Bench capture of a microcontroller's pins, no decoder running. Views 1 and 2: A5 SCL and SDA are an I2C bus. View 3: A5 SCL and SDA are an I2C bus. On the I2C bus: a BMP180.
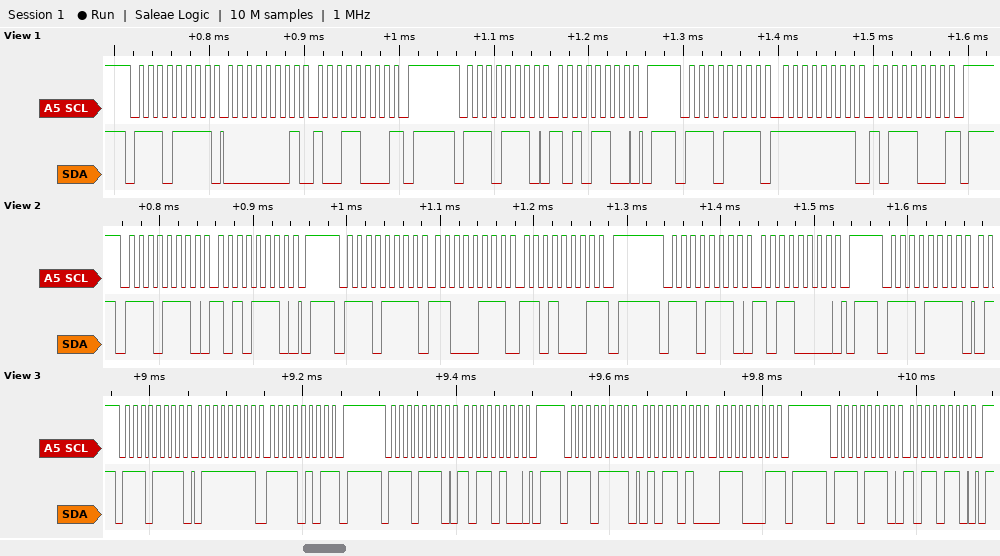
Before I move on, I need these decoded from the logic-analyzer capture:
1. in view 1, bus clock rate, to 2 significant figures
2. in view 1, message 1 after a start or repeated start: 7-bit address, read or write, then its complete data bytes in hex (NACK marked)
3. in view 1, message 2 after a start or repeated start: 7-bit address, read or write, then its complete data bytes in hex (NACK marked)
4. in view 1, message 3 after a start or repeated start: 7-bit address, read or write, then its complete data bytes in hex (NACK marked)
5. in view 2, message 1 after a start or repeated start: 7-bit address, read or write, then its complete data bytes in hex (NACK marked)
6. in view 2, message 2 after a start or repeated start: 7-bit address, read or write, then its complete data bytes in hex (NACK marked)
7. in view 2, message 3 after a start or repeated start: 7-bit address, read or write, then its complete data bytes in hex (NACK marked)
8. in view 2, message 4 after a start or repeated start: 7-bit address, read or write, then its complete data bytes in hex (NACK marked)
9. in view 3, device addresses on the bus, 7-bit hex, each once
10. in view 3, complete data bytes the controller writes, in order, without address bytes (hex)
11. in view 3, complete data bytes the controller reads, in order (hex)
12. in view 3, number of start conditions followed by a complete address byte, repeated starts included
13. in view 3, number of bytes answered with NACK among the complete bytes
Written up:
100 kHz
0x77 read: 01 98 NACK
0x77 write: AC
0x77 read: FF B8 NACK
0x77 write: AE
0x77 read: C7 D1 NACK
0x77 write: B0
0x77 read
0x77
B4 B6
7F F5 5A 71
4
2
